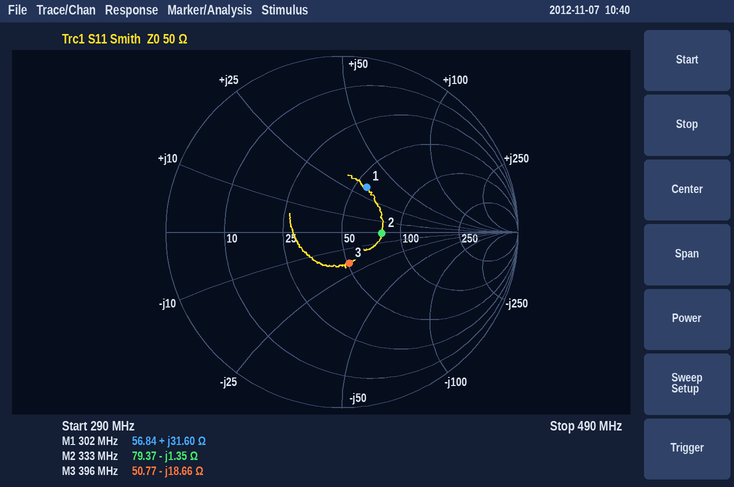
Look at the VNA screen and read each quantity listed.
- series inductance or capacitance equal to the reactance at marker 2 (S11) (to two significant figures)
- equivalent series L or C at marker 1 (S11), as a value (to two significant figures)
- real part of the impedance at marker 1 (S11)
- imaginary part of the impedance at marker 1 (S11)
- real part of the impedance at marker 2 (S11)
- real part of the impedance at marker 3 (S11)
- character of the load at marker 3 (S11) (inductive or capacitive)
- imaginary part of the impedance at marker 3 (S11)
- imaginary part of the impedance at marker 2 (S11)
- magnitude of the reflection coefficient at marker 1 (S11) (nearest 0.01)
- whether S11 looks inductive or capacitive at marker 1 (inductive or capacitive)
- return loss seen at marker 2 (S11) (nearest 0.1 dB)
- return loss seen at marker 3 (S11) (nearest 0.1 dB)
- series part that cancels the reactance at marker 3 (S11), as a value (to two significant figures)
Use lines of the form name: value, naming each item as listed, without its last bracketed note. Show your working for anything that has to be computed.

series inductance or capacitance equal to the reactance at marker 2 (S11): C = 1/(2π × 333 MHz × 1.35 Ω) ≈ 354 pF, so 350 pF to two significant figures
equivalent series L or C at marker 1 (S11), as a value: L = 31.6 Ω/(2π × 302 MHz) ≈ 17 nH
real part of the impedance at marker 1: 56.84 Ω
imaginary part of the impedance at marker 1: +31.60 Ω
real part of the impedance at marker 2: 79.37 Ω
real part of the impedance at marker 3: 50.77 Ω
character of the load at marker 3 (S11): capacitive
imaginary part of the impedance at marker 3: -18.66 Ω
imaginary part of the impedance at marker 2: -1.35 Ω
magnitude of the reflection coefficient at marker 1 (S11): 0.29
whether S11 looks inductive or capacitive at marker 1: inductive
return loss seen at marker 2 (S11): 12.9 dB
return loss seen at marker 3 (S11): 14.8 dB
series part that cancels the reactance at marker 3 (S11), as a value: L = 18.66 Ω/(2π × 396 MHz) ≈ 7.5 nH
